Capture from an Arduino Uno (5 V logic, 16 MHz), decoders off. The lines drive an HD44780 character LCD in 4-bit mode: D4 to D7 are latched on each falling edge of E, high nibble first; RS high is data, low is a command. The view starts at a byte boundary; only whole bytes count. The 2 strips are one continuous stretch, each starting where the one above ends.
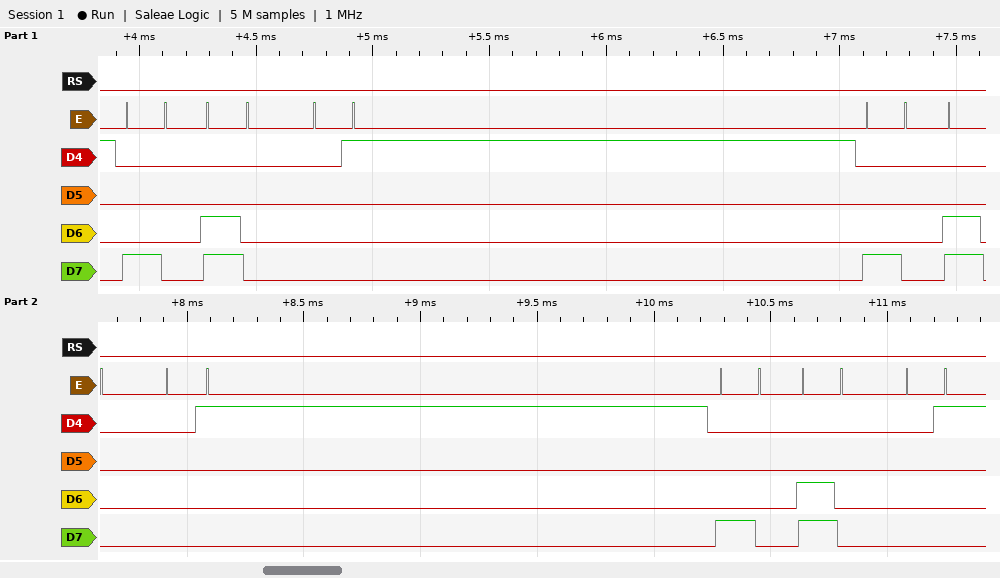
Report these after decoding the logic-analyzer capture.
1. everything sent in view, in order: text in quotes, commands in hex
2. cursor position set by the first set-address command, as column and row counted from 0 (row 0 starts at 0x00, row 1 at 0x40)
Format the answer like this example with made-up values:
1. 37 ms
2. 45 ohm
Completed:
1. 0x80 0xC0 0x01 0x80 0xC0 0x01 0x80 0xC0 0x01
2. column 0, row 0
